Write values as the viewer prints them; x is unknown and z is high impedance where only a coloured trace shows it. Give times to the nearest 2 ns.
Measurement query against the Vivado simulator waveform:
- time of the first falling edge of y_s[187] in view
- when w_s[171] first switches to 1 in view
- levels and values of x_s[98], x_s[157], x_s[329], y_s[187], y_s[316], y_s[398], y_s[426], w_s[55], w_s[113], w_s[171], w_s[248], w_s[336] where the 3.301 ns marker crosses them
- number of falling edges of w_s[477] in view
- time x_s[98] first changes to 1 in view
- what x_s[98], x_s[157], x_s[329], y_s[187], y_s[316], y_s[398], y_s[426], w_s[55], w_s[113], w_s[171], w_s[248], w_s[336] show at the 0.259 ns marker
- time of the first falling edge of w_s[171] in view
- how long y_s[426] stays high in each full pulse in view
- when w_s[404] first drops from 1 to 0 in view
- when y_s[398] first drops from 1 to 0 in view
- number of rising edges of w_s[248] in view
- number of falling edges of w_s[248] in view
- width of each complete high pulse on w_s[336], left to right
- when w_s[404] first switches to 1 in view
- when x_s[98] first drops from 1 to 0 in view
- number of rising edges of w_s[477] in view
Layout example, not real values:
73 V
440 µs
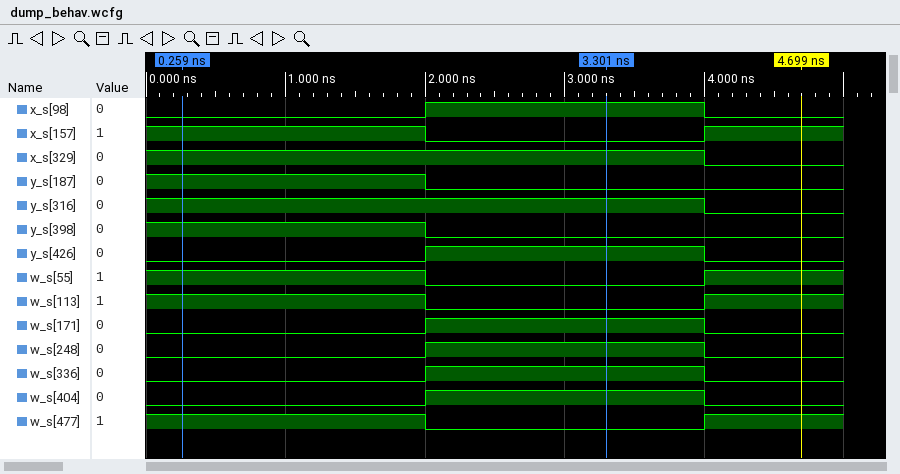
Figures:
2 ns
2 ns
x_s[98]=1, x_s[157]=0, x_s[329]=1, y_s[187]=0, y_s[316]=1, y_s[398]=0, y_s[426]=1, w_s[55]=0, w_s[113]=0, w_s[171]=1, w_s[248]=1, w_s[336]=1
1
2 ns
x_s[98]=0, x_s[157]=1, x_s[329]=1, y_s[187]=1, y_s[316]=1, y_s[398]=1, y_s[426]=0, w_s[55]=1, w_s[113]=1, w_s[171]=0, w_s[248]=0, w_s[336]=0
4 ns
2 ns
4 ns
2 ns
1
1
2 ns
2 ns
4 ns
1
